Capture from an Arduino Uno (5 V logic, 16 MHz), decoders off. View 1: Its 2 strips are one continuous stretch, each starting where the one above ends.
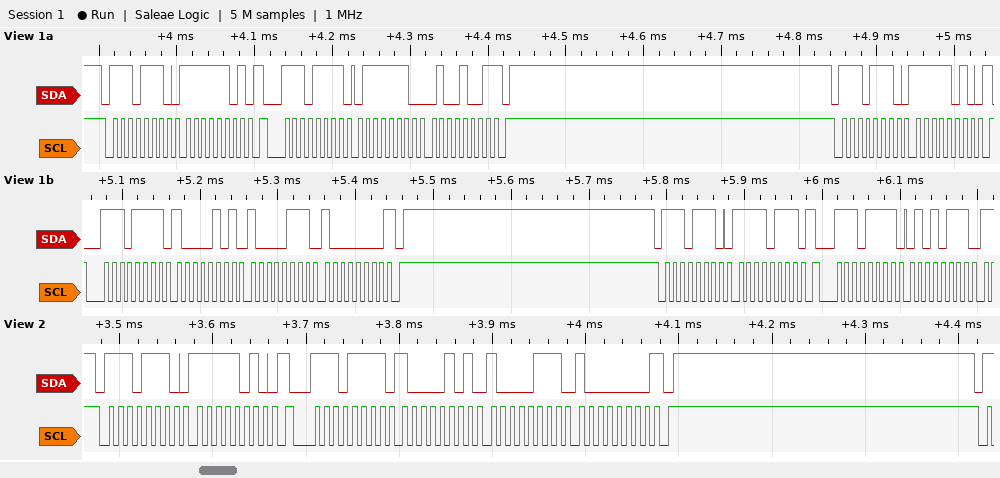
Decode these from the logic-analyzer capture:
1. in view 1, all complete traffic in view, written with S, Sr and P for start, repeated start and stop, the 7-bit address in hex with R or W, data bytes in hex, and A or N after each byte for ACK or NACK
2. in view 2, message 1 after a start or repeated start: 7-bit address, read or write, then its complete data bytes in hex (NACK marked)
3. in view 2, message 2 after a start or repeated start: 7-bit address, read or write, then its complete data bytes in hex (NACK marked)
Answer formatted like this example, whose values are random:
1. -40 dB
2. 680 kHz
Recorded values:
1. S 77W A FD A Sr 77R A 7E A 49 N P S 77W A FA A Sr 77R A 85 A 87 A 80 N P S 77W A F7 A Sr 77R A 57 A
2. 0x77 write: FA
3. 0x77 read: 85 87 80 NACK
